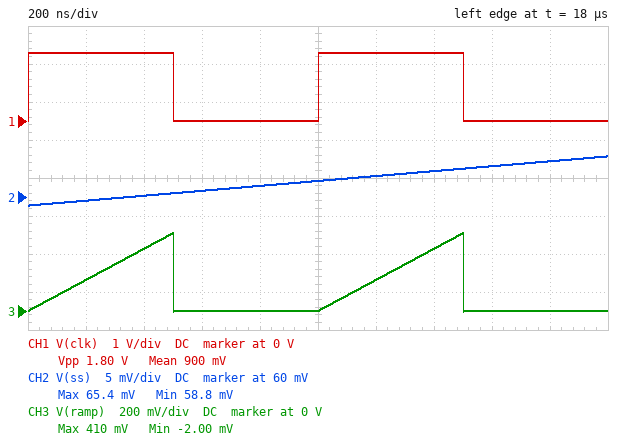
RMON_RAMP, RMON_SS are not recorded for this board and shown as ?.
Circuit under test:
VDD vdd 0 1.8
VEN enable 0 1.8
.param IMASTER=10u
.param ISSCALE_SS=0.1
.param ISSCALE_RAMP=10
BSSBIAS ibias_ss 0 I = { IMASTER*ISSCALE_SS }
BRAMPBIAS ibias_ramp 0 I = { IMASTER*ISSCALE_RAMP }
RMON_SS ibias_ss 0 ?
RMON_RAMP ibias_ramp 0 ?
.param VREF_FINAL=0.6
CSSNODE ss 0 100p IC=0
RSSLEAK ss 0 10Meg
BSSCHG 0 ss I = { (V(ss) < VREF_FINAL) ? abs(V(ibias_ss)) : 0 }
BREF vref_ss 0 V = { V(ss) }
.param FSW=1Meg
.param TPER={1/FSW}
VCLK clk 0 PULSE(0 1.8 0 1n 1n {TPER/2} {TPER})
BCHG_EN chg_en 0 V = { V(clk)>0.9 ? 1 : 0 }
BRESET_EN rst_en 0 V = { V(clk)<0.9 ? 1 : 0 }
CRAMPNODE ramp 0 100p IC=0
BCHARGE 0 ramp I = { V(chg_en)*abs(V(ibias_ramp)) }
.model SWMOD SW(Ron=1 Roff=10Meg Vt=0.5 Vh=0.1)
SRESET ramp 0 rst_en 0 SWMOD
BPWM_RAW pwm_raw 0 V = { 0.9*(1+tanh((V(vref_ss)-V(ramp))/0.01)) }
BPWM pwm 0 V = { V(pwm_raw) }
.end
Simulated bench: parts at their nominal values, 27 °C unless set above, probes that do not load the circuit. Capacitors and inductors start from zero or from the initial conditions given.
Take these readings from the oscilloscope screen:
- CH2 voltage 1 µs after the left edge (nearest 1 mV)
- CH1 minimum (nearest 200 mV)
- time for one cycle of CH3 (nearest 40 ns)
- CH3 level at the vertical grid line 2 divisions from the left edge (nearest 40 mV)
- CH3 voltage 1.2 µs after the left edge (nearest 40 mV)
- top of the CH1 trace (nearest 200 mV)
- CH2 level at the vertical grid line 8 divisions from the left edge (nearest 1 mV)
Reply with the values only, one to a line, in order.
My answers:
62 mV
0 V
1.00 µs
320 mV
160 mV
1.8 V
64 mV
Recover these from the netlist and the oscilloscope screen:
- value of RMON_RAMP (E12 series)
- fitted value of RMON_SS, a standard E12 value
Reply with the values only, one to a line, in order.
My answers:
0.82 Ω
0.33 Ω
